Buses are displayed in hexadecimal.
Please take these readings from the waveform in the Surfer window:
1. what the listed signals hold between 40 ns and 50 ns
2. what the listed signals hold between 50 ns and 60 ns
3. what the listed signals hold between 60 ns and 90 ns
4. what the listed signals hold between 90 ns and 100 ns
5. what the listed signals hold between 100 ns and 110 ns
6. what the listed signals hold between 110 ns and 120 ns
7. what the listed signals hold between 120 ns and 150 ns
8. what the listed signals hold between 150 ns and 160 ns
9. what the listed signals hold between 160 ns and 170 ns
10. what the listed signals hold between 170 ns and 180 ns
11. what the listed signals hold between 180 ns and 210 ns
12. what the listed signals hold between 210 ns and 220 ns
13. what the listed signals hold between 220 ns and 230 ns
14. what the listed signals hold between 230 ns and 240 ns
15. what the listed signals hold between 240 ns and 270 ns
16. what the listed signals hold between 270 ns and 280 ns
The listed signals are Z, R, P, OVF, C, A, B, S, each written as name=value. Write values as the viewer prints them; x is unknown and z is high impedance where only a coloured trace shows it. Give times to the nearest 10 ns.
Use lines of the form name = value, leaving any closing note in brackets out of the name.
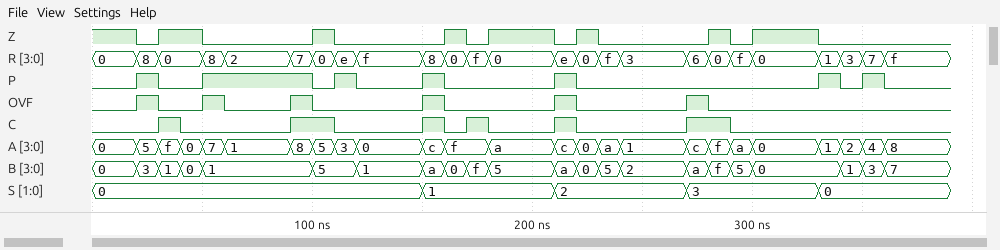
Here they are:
what the listed signals hold between 40 ns and 50 ns = Z=1, R=0, P=0, OVF=0, C=0, A=0, B=0, S=0
what the listed signals hold between 50 ns and 60 ns = Z=0, R=8, P=1, OVF=1, C=0, A=7, B=1, S=0
what the listed signals hold between 60 ns and 90 ns = Z=0, R=2, P=1, OVF=0, C=0, A=1, B=1, S=0
what the listed signals hold between 90 ns and 100 ns = Z=0, R=7, P=1, OVF=1, C=1, A=8, B=1, S=0
what the listed signals hold between 100 ns and 110 ns = Z=1, R=0, P=0, OVF=0, C=1, A=5, B=5, S=0
what the listed signals hold between 110 ns and 120 ns = Z=0, R=e, P=1, OVF=0, C=0, A=3, B=5, S=0
what the listed signals hold between 120 ns and 150 ns = Z=0, R=f, P=0, OVF=0, C=0, A=0, B=1, S=0
what the listed signals hold between 150 ns and 160 ns = Z=0, R=8, P=1, OVF=1, C=1, A=c, B=a, S=1
what the listed signals hold between 160 ns and 170 ns = Z=1, R=0, P=0, OVF=0, C=0, A=f, B=0, S=1
what the listed signals hold between 170 ns and 180 ns = Z=0, R=f, P=0, OVF=0, C=1, A=f, B=f, S=1
what the listed signals hold between 180 ns and 210 ns = Z=1, R=0, P=0, OVF=0, C=0, A=a, B=5, S=1
what the listed signals hold between 210 ns and 220 ns = Z=0, R=e, P=1, OVF=1, C=1, A=c, B=a, S=2
what the listed signals hold between 220 ns and 230 ns = Z=1, R=0, P=0, OVF=0, C=0, A=0, B=0, S=2
what the listed signals hold between 230 ns and 240 ns = Z=0, R=f, P=0, OVF=0, C=0, A=a, B=5, S=2
what the listed signals hold between 240 ns and 270 ns = Z=0, R=3, P=0, OVF=0, C=0, A=1, B=2, S=2
what the listed signals hold between 270 ns and 280 ns = Z=0, R=6, P=0, OVF=1, C=1, A=c, B=a, S=3
